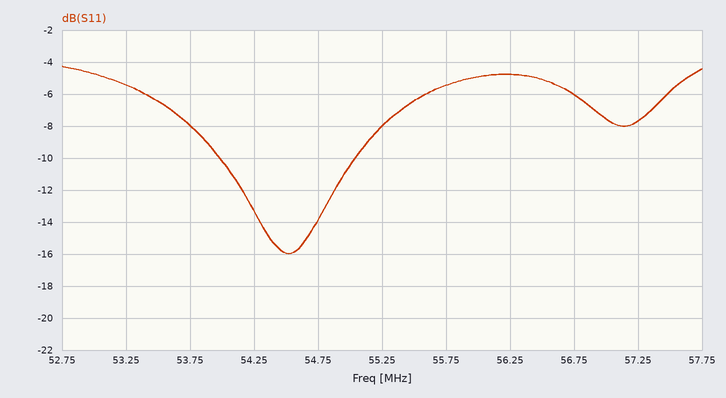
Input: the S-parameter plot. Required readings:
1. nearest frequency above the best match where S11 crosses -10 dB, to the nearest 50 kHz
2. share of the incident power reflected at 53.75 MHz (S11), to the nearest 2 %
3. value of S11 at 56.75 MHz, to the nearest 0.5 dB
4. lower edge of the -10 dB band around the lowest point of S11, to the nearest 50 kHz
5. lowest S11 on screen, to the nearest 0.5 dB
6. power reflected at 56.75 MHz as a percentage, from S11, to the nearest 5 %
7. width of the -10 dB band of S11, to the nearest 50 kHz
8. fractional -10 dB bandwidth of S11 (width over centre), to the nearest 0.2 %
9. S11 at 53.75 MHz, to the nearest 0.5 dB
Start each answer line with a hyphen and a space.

- 55.05 MHz
- 16 %
- -6.0 dB
- 54.00 MHz
- -16.0 dB
- 25 %
- 1.05 MHz
- 2.0 %
- -8.0 dB
